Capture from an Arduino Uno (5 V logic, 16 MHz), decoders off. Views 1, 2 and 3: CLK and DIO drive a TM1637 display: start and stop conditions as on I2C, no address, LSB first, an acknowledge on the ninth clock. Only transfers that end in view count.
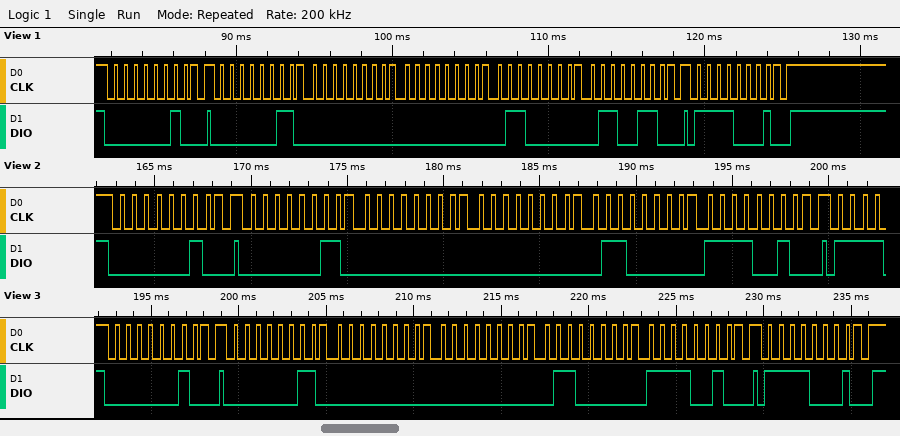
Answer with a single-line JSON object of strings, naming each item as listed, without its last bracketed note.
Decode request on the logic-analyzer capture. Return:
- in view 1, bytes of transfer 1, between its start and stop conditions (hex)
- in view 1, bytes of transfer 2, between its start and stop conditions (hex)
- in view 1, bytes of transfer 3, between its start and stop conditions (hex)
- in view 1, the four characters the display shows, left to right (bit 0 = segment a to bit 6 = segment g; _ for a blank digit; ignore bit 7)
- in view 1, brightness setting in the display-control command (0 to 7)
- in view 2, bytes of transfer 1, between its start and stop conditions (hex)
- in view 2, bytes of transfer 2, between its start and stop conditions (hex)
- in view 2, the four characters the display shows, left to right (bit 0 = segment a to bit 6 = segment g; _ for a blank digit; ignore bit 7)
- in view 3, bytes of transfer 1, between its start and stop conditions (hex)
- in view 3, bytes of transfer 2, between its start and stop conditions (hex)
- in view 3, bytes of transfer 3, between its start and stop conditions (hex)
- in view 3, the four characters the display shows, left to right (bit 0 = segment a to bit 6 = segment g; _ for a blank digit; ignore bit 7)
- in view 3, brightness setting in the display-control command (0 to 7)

{"in view 1, bytes of transfer 1, between its start and stop conditions": "40", "in view 1, bytes of transfer 2, between its start and stop conditions": "C0 00 00 06 66", "in view 1, bytes of transfer 3, between its start and stop conditions": "8F", "in view 1, the four characters the display shows, left to right": "__14", "in view 1, brightness setting in the display-control command": "7", "in view 2, bytes of transfer 1, between its start and stop conditions": "40", "in view 2, bytes of transfer 2, between its start and stop conditions": "C0 00 00 06 4F", "in view 2, the four characters the display shows, left to right": "__13", "in view 3, bytes of transfer 1, between its start and stop conditions": "40", "in view 3, bytes of transfer 2, between its start and stop conditions": "C0 00 00 06 4F", "in view 3, bytes of transfer 3, between its start and stop conditions": "8F", "in view 3, the four characters the display shows, left to right": "__13", "in view 3, brightness setting in the display-control command": "7"}
